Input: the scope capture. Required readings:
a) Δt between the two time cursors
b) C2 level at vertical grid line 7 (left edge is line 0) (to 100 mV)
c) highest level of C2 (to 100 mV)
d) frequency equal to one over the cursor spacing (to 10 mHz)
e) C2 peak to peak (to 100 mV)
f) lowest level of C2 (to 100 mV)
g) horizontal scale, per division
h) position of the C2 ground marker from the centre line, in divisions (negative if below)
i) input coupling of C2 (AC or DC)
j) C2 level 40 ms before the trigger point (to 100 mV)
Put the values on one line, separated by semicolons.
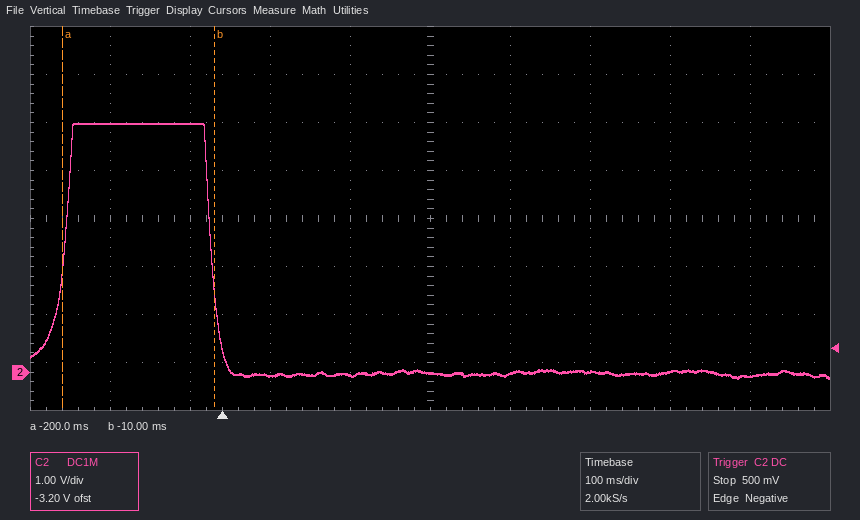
190 ms; 0.0 V; 5.2 V; 5.26 Hz; 5.3 V; -100 mV; 100 ms; -3.2 div; DC; 5.2 V
